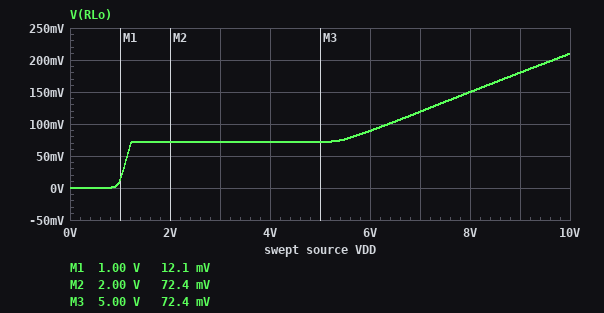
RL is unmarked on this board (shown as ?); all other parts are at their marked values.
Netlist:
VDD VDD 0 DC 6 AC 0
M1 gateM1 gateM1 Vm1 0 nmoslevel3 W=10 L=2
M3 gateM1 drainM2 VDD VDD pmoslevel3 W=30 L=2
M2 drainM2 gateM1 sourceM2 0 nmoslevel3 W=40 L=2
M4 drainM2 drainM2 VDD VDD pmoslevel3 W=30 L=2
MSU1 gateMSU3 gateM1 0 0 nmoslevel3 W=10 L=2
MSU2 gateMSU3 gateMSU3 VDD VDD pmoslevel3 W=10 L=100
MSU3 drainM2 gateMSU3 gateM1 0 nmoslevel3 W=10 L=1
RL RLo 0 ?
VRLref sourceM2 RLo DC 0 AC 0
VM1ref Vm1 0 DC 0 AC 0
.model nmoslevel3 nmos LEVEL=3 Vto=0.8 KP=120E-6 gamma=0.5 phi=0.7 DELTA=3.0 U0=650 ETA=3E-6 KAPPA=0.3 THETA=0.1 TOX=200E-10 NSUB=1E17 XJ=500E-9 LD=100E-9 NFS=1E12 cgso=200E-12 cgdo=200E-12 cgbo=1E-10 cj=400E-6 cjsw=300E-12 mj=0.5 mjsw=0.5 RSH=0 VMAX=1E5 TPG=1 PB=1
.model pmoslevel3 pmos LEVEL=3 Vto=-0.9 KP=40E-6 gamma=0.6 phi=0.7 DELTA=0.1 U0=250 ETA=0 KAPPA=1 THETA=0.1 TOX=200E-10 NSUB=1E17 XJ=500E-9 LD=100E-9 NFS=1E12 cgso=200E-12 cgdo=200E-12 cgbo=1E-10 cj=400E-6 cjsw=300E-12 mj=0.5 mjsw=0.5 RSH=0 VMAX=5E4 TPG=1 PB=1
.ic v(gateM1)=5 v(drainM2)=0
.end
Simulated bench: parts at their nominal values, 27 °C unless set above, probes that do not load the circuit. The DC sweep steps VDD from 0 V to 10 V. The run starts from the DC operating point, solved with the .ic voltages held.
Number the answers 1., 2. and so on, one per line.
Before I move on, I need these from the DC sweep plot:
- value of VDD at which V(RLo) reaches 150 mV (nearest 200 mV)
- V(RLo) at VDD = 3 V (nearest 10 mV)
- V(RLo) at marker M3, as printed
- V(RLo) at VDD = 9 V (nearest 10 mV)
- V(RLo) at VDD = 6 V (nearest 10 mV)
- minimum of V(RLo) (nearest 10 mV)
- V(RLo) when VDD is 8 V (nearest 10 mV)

1. 8.0 V
2. 70 mV
3. 72.4 mV
4. 180 mV
5. 90 mV
6. 0 V
7. 150 mV
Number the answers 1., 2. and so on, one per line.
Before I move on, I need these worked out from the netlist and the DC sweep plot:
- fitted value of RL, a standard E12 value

1. 8.2 kΩ
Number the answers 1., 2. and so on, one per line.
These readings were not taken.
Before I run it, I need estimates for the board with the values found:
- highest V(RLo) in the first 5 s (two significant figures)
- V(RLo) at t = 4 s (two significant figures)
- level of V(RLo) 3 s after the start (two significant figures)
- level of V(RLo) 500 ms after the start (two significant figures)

1. 44 mV
2. 33 mV
3. 23 mV
4. 3.0 mV
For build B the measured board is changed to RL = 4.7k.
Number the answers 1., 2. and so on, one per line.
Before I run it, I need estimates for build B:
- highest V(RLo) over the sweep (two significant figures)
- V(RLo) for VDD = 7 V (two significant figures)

1. 180 mV
2. 130 mV
